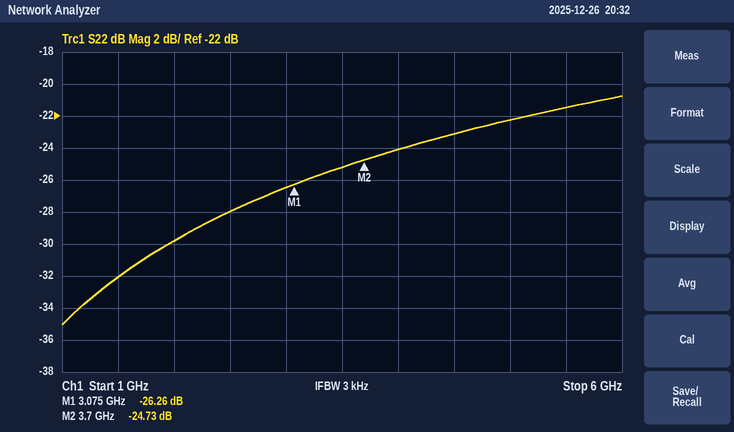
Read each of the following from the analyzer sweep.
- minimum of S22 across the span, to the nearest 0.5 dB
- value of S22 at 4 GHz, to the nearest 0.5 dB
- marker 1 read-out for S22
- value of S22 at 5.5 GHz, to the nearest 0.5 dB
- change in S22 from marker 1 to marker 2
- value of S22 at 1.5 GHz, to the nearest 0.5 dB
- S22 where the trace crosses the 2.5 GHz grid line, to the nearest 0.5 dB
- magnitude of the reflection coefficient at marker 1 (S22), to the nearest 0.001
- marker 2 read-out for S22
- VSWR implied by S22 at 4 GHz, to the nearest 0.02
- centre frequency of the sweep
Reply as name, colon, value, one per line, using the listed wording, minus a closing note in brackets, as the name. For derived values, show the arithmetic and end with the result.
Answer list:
minimum of S22 across the span, to the nearest 0.5 dB: -35.0 dB
value of S22 at 4 GHz, to the nearest 0.5 dB: -24.0 dB
marker 1 read-out for S22: -26.26 dB
value of S22 at 5.5 GHz, to the nearest 0.5 dB: -21.5 dB
change in S22 from marker 1 to marker 2: -24.73 − (-26.26) = 1.53 dB
value of S22 at 1.5 GHz, to the nearest 0.5 dB: -32.0 dB
S22 where the trace crosses the 2.5 GHz grid line, to the nearest 0.5 dB: -28.0 dB
magnitude of the reflection coefficient at marker 1 (S22), to the nearest 0.001: 10^(-26.26/20) ≈ 0.049
marker 2 read-out for S22: -24.73 dB
VSWR implied by S22 at 4 GHz, to the nearest 0.02: |Γ| = 10^(-24/20) = 0.0631; VSWR = (1 + 0.0631)/(1 − 0.0631) ≈ 1.13, so 1.14 to the nearest 0.02
centre frequency of the sweep: 3.5 GHz
